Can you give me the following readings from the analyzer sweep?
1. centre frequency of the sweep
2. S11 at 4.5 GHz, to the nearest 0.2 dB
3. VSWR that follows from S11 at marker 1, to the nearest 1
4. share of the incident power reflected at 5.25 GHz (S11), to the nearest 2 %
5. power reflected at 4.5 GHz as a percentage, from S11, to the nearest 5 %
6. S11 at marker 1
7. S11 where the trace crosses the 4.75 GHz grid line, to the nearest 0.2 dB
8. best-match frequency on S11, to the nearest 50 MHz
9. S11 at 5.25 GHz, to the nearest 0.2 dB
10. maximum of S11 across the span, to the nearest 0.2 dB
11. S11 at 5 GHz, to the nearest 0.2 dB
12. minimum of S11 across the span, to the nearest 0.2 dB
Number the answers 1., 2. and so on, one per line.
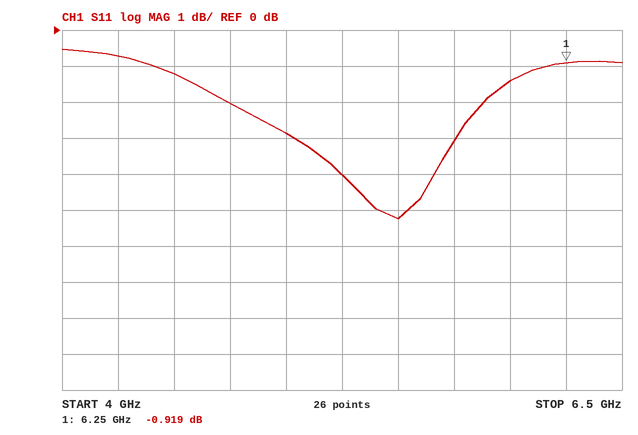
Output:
1. 5.25 GHz
2. -1.2 dB
3. 19
4. 40 %
5. 75 %
6. -0.919 dB
7. -2.0 dB
8. 5.50 GHz
9. -4.0 dB
10. -0.6 dB
11. -2.8 dB
12. -5.2 dB
